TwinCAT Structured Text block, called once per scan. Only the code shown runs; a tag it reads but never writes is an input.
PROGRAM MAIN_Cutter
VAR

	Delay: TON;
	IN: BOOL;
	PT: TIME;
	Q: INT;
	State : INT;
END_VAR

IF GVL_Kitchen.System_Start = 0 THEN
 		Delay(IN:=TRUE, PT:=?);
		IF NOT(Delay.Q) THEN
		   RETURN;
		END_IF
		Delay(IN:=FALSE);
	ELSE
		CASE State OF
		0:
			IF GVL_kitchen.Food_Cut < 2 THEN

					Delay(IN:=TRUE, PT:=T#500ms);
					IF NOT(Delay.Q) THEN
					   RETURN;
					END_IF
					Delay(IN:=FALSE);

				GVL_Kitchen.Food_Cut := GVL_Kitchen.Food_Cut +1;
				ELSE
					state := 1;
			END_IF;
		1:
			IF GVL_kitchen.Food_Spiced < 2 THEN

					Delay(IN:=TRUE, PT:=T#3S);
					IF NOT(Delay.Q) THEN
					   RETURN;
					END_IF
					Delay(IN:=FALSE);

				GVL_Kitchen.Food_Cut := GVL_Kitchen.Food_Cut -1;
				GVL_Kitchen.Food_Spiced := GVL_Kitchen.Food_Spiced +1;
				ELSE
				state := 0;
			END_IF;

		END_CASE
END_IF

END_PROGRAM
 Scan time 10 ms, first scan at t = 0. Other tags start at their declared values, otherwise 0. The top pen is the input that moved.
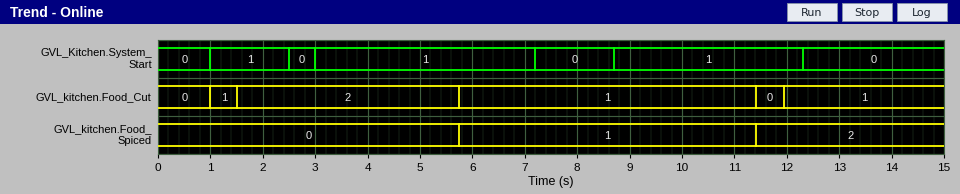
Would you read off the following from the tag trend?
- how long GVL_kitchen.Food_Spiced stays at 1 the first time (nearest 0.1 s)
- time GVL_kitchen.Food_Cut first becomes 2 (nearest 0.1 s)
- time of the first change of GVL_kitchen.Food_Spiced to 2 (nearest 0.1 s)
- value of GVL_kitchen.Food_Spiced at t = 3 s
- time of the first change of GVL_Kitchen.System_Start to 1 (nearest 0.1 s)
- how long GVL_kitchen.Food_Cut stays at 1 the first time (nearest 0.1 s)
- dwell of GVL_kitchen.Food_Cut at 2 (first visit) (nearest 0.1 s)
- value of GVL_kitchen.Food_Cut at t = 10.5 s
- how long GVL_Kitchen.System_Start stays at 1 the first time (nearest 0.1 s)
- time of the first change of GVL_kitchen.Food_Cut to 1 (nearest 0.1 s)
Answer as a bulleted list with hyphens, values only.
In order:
- 5.7 s
- 1.5 s
- 11.4 s
- 0
- 1.0 s
- 0.5 s
- 4.2 s
- 1
- 1.5 s
- 1.0 s
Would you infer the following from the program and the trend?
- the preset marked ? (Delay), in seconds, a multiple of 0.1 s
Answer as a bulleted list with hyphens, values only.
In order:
- 1.2 s
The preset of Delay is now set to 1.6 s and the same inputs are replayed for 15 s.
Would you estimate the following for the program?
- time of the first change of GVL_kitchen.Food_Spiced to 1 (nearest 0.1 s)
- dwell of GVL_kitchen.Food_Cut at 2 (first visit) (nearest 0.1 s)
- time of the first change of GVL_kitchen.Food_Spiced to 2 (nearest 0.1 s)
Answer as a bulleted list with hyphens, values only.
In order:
- 4.5 s
- 3.0 s
- 10.2 s
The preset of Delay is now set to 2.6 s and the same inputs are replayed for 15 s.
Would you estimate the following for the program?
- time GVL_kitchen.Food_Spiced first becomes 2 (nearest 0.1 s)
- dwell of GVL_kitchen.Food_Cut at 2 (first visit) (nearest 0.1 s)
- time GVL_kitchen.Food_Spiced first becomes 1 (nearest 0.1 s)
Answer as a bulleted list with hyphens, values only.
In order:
- 10.2 s
- 3.0 s
- 4.5 s
